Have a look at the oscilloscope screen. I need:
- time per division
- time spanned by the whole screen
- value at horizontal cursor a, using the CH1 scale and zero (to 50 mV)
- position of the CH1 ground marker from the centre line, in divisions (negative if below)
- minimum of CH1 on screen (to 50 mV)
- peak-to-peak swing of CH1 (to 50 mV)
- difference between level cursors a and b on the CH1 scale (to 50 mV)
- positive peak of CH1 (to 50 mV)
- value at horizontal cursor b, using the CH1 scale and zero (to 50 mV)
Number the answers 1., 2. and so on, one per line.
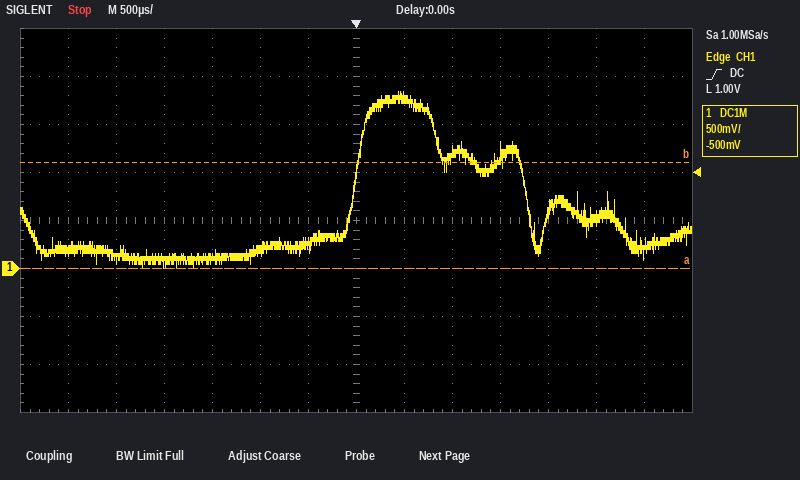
1. 500 µs
2. 7 ms
3. 0 mV
4. -1.0 div
5. 0 mV
6. 1.85 V
7. 1.10 V
8. 1.85 V
9. 1.10 V
